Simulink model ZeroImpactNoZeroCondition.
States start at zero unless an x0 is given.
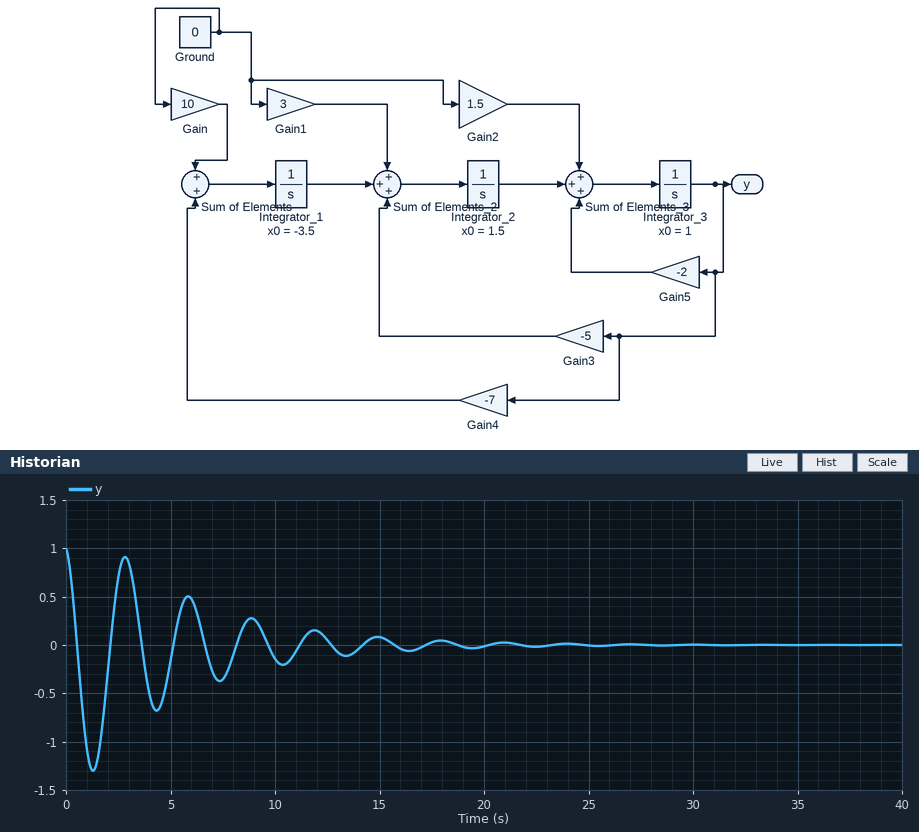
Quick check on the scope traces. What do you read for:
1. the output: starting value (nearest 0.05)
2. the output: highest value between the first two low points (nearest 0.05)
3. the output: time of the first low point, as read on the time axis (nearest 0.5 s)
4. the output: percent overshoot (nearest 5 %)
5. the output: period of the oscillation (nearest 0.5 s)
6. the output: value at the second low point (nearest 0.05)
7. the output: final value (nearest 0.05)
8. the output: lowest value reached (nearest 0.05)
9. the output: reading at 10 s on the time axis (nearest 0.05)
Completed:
1.00
0.90
1.5 s
130 %
3.0 s
-0.70
0.00
-1.30
-0.15
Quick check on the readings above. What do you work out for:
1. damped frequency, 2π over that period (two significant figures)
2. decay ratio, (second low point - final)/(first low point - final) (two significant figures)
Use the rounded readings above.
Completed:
2.1 rad/s
0.54
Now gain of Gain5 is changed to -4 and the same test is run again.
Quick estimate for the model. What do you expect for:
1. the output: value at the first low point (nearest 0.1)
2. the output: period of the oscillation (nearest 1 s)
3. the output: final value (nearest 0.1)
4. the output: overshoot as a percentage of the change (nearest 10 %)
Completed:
-0.7
4 s
0.0
70 %
